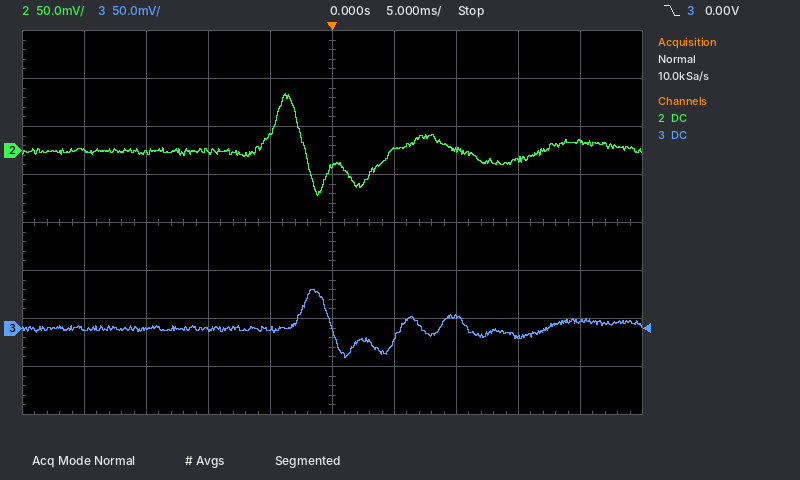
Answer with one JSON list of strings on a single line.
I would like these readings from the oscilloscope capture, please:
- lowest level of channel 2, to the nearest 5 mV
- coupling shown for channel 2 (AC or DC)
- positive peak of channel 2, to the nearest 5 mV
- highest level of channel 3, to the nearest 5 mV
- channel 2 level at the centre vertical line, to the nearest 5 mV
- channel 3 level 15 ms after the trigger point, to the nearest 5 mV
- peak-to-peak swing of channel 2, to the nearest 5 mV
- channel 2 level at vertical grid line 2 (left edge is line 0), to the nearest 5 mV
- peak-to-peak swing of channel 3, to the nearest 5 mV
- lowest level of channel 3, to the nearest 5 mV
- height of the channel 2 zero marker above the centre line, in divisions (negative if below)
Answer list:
["-45 mV", "DC", "60 mV", "40 mV", "-15 mV", "-10 mV", "105 mV", "0 mV", "70 mV", "-30 mV", "+1.5 div"]
